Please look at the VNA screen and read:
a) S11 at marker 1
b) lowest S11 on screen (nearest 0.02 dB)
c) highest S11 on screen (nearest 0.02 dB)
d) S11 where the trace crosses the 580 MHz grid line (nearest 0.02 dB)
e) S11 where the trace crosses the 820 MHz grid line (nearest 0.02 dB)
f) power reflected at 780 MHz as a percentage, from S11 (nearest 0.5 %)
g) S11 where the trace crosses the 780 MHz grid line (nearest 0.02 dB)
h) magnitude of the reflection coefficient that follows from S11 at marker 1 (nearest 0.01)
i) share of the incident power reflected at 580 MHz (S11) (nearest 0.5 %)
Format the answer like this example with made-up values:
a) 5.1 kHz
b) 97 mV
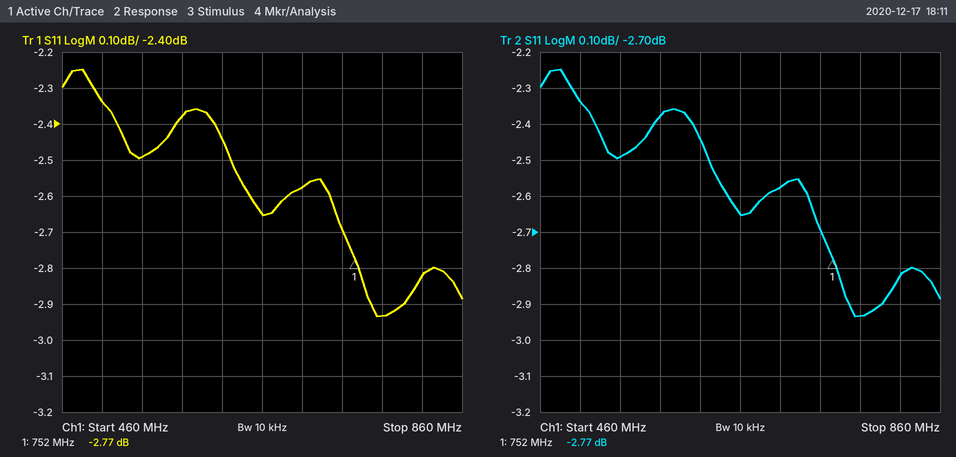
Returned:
a) -2.77 dB
b) -2.94 dB
c) -2.24 dB
d) -2.38 dB
e) -2.82 dB
f) 51.0 %
g) -2.94 dB
h) 0.73
i) 58.0 %
